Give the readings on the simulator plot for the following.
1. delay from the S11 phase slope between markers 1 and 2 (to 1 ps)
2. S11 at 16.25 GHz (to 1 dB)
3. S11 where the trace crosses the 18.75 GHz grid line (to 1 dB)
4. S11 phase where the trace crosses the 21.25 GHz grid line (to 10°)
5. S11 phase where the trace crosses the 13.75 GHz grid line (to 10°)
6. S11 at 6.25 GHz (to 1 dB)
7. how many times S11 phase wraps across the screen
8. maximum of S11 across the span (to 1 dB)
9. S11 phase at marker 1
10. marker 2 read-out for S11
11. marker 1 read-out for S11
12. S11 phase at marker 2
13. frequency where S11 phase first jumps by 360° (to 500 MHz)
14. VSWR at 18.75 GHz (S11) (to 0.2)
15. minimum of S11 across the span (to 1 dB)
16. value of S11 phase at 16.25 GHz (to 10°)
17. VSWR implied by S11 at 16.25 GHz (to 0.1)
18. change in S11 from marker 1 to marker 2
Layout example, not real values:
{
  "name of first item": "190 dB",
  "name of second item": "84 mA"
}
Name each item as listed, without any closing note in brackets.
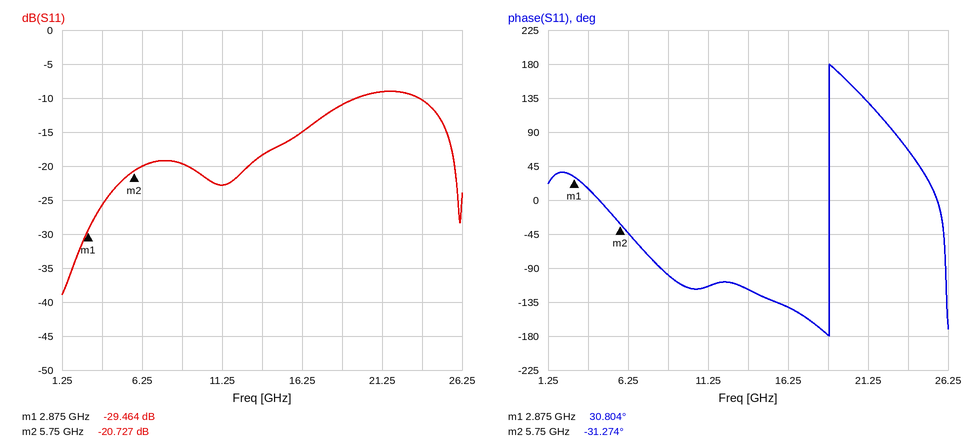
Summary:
{
  "delay from the S11 phase slope between markers 1 and 2": "60 ps",
  "S11 at 16.25 GHz": "-15 dB",
  "S11 where the trace crosses the 18.75 GHz grid line": "-11 dB",
  "S11 phase where the trace crosses the 21.25 GHz grid line": "130°",
  "S11 phase where the trace crosses the 13.75 GHz grid line": "-120°",
  "S11 at 6.25 GHz": "-20 dB",
  "how many times S11 phase wraps across the screen": "1",
  "maximum of S11 across the span": "-9 dB",
  "S11 phase at marker 1": "30.804°",
  "marker 2 read-out for S11": "-20.727 dB",
  "marker 1 read-out for S11": "-29.464 dB",
  "S11 phase at marker 2": "-31.274°",
  "frequency where S11 phase first jumps by 360°": "19.0 GHz",
  "VSWR at 18.75 GHz (S11)": "1.8",
  "minimum of S11 across the span": "-39 dB",
  "value of S11 phase at 16.25 GHz": "-140°",
  "VSWR implied by S11 at 16.25 GHz": "1.4",
  "change in S11 from marker 1 to marker 2": "8.737 dB"
}
